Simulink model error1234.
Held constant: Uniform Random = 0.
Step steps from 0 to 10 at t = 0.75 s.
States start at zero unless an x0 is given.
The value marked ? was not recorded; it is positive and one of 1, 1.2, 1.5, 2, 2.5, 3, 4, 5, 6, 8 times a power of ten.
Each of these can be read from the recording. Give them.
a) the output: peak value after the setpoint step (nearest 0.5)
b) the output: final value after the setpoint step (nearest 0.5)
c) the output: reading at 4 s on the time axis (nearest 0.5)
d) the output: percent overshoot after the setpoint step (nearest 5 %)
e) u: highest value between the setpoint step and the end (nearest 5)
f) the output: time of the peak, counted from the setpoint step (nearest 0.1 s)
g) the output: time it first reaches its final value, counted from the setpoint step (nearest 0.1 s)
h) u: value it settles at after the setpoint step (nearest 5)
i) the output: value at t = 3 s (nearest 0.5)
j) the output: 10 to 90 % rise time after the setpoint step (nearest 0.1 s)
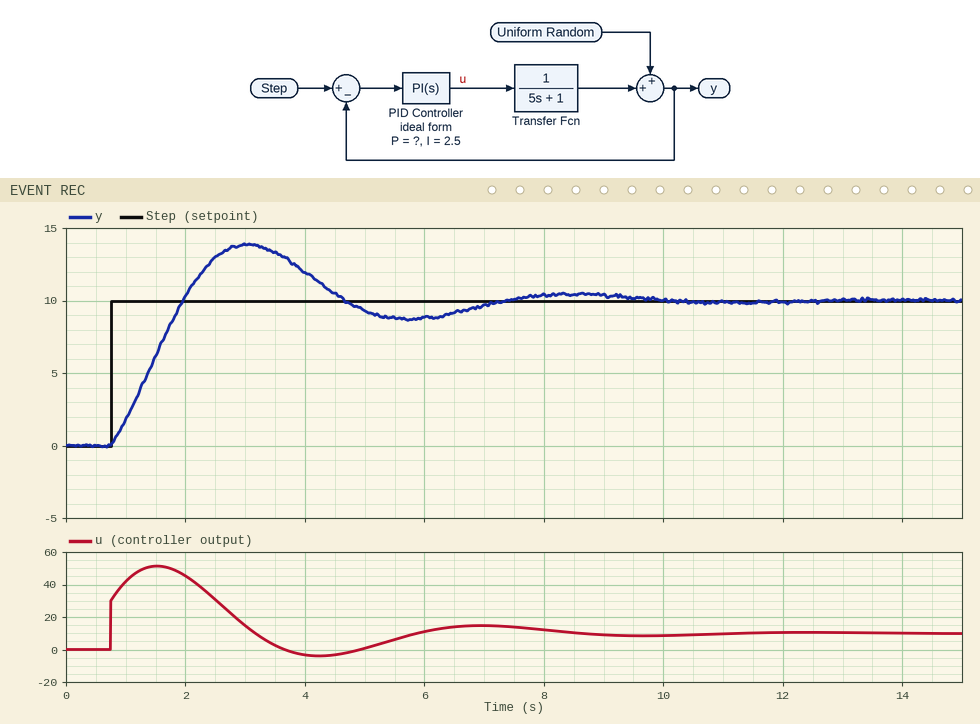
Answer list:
14.0
10.0
12.0
40 %
50
2.3 s
1.2 s
10
14.0
0.9 s
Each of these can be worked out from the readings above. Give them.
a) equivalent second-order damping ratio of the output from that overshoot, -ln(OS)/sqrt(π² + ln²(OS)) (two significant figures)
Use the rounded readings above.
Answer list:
0.28
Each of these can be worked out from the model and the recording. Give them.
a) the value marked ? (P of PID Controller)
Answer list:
3
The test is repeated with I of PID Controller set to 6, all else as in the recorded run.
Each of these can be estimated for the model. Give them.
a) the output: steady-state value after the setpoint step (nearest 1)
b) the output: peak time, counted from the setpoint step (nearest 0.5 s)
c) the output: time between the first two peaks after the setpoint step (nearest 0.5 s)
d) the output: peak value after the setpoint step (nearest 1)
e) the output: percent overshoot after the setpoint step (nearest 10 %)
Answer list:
10
1.5 s
3.5 s
15
50 %
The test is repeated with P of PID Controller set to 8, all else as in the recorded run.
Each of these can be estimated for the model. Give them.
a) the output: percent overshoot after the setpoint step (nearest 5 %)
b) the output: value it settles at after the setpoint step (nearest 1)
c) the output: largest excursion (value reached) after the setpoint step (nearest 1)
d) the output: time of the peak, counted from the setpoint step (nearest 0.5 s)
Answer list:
30 %
10
13
1.5 s
